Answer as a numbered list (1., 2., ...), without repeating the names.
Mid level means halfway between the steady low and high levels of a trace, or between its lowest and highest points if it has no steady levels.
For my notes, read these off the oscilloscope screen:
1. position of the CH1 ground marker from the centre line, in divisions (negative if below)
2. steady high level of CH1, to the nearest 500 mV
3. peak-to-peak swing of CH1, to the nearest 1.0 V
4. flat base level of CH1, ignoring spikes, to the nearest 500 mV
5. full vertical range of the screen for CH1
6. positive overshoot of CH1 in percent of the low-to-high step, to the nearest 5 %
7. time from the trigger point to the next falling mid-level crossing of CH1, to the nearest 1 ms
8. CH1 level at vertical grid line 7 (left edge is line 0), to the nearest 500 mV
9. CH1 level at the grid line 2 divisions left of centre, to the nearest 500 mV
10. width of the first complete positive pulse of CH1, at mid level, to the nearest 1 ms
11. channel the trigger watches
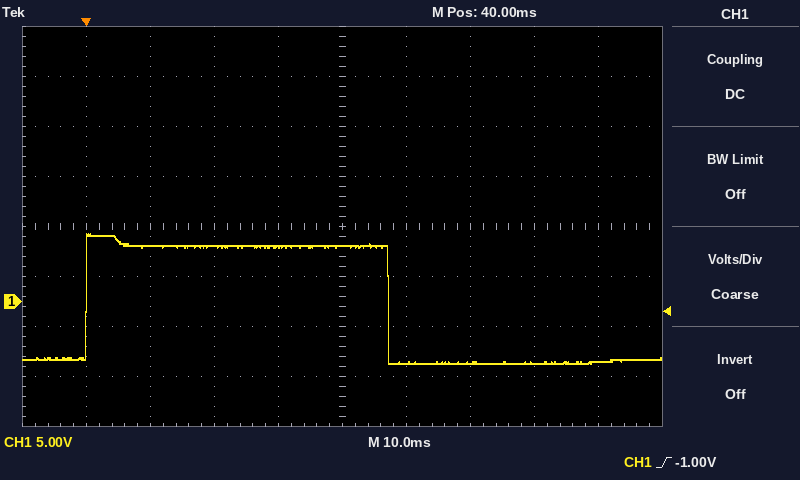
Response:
1. -1.5 div
2. 5.5 V
3. 13.0 V
4. -6.0 V
5. 40 V
6. 10 %
7. 47 ms
8. -6.0 V
9. 5.5 V
10. 47 ms
11. CH1
